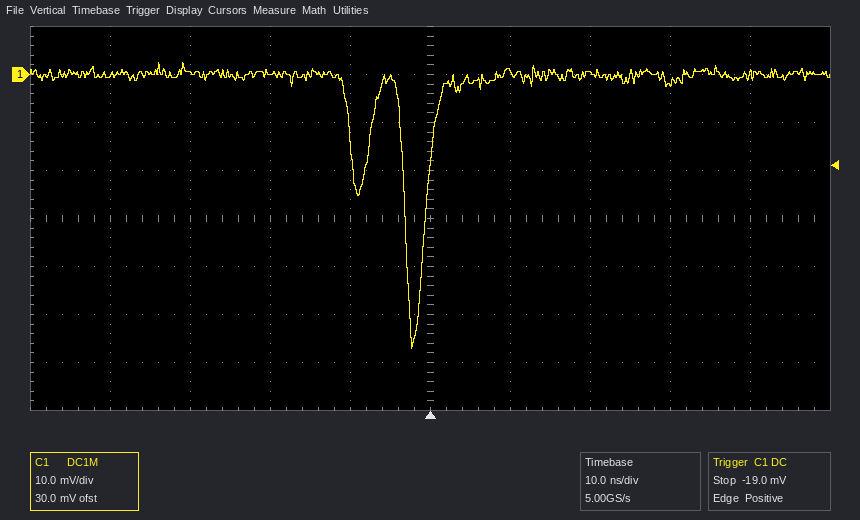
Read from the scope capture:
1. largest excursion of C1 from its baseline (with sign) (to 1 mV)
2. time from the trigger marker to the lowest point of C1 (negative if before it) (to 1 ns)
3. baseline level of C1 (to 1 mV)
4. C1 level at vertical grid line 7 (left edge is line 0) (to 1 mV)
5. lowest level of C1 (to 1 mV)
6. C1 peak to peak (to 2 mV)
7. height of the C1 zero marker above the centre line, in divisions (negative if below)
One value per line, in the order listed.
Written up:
-57 mV
-2 ns
0 mV
0 mV
-57 mV
60 mV
+3.0 div
